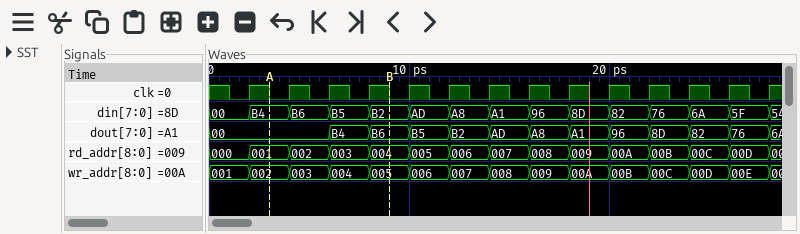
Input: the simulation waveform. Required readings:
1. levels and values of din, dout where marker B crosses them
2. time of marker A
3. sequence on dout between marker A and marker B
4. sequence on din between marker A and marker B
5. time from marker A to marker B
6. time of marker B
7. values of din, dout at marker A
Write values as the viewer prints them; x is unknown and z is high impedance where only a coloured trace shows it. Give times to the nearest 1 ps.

din=B2, dout=B6
3 ps
00, B4, B6
B4, B6, B5, B2
6 ps
9 ps
din=B4, dout=00
